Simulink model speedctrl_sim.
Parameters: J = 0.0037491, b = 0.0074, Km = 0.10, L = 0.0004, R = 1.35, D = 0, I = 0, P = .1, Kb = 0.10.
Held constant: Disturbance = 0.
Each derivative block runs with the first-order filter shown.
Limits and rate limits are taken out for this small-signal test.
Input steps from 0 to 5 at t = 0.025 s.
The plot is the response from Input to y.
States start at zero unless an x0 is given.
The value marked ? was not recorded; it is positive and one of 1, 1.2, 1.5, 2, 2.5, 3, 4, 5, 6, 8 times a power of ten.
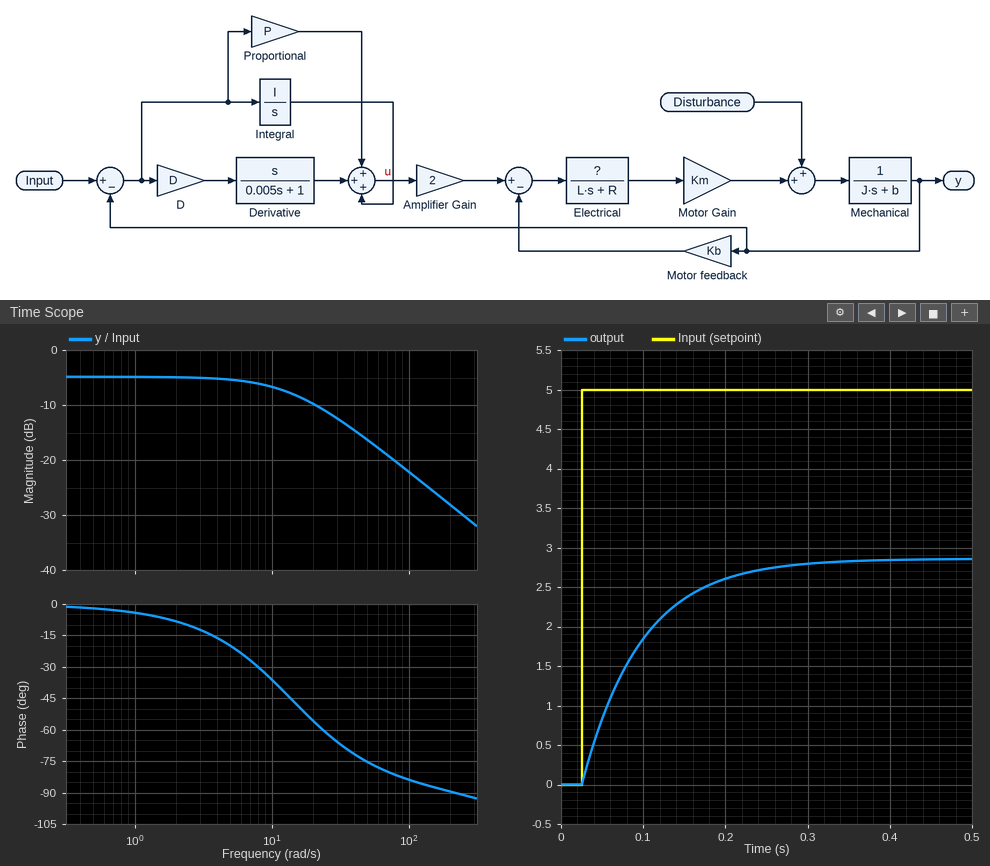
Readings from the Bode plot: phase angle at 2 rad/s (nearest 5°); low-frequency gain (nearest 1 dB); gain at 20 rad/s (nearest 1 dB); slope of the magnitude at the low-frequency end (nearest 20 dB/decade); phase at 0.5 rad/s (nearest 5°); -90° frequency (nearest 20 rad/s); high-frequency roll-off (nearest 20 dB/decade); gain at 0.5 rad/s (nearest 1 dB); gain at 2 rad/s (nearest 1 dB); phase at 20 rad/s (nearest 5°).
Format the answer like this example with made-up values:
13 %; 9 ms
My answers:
-10°; -5 dB; -10 dB; 0 dB/decade; 0°; 220 rad/s; -20 dB/decade; -5 dB; -5 dB; -55°
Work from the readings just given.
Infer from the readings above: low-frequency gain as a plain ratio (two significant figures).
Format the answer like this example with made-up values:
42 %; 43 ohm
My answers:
0.56
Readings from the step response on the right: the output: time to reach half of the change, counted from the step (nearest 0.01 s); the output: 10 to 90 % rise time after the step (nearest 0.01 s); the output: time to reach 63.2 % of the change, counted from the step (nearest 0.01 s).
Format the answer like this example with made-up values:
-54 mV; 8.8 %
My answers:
0.05 s; 0.16 s; 0.07 s
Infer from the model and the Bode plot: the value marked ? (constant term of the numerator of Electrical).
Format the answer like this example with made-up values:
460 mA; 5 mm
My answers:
2
